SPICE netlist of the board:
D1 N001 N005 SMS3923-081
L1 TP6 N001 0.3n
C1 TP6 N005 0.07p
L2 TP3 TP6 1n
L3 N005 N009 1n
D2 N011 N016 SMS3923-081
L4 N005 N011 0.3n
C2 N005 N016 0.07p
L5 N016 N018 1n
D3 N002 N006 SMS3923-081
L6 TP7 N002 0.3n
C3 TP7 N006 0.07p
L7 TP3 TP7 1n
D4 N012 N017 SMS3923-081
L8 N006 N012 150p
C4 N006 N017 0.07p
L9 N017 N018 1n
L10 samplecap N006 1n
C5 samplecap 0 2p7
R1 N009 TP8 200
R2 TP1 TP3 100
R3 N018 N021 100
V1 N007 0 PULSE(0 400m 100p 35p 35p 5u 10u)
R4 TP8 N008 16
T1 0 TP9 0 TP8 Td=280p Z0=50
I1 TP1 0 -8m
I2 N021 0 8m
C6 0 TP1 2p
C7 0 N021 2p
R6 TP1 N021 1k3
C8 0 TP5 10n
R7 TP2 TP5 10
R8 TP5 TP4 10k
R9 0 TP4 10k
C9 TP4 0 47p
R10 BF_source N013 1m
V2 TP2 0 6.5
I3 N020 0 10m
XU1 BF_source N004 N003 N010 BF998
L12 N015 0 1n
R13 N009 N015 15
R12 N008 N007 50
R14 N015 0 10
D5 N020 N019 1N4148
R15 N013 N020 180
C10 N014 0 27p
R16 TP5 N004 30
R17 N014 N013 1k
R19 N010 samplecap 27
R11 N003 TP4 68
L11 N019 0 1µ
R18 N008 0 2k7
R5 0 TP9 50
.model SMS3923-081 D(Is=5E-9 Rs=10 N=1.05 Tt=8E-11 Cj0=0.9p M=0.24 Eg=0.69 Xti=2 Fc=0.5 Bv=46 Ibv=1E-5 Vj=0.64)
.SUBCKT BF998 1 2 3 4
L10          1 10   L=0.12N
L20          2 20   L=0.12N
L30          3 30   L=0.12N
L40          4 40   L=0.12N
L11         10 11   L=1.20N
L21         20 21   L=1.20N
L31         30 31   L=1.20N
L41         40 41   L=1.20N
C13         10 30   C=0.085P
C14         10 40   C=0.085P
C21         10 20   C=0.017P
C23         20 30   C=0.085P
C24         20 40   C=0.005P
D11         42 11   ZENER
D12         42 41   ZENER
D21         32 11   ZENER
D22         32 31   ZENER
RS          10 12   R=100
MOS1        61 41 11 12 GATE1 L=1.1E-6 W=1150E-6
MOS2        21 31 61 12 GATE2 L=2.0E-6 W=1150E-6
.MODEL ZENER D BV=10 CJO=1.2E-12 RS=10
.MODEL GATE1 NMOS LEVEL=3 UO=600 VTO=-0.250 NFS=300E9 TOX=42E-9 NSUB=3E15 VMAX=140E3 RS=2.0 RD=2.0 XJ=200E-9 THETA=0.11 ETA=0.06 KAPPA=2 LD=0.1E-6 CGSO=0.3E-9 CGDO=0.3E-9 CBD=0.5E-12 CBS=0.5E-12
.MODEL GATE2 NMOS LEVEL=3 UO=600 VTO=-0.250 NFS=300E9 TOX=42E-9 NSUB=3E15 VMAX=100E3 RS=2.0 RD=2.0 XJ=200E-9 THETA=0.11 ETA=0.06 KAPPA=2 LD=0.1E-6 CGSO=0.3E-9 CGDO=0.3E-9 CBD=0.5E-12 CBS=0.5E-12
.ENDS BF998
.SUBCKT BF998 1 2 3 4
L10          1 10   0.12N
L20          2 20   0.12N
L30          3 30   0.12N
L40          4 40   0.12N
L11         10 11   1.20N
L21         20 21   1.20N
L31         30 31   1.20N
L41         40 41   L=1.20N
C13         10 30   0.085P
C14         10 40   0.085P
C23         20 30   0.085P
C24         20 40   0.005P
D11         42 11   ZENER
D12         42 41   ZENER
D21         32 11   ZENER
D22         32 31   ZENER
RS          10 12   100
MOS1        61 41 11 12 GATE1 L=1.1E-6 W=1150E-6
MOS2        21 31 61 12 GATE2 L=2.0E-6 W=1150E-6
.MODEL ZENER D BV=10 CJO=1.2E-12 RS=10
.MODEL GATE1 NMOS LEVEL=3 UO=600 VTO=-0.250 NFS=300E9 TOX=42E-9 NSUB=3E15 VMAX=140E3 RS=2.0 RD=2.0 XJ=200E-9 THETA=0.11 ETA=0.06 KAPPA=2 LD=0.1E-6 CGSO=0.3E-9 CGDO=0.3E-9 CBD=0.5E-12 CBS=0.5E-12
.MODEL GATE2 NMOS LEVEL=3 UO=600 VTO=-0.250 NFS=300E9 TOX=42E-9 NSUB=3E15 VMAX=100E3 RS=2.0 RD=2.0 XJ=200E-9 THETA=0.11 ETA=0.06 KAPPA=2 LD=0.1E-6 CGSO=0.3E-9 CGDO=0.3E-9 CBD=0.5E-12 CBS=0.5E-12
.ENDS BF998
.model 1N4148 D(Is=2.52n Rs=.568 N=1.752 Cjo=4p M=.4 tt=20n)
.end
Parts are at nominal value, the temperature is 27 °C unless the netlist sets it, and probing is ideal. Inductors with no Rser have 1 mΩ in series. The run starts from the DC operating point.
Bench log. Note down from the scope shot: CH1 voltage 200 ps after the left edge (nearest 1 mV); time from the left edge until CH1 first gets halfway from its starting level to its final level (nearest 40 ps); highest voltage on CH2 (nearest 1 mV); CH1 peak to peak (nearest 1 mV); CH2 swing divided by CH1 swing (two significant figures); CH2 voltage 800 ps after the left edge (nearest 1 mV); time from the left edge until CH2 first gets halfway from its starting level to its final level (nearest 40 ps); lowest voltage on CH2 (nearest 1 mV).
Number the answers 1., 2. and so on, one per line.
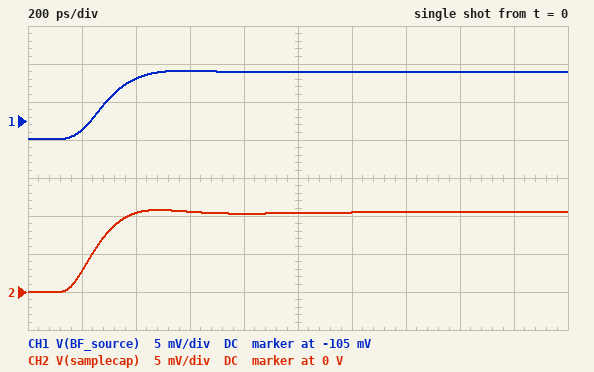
1. -106 mV
2. 280 ps
3. 11 mV
4. 9 mV
5. 1.2
6. 10 mV
7. 240 ps
8. 0 V
